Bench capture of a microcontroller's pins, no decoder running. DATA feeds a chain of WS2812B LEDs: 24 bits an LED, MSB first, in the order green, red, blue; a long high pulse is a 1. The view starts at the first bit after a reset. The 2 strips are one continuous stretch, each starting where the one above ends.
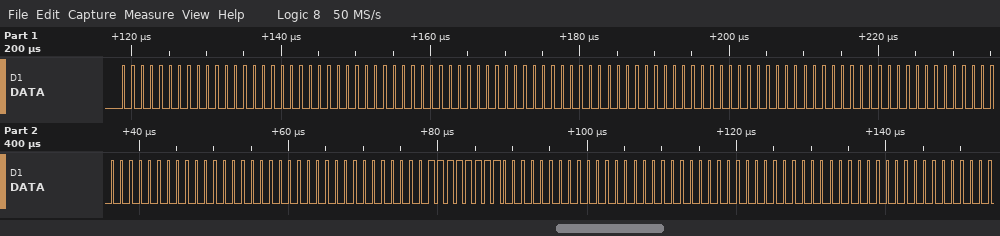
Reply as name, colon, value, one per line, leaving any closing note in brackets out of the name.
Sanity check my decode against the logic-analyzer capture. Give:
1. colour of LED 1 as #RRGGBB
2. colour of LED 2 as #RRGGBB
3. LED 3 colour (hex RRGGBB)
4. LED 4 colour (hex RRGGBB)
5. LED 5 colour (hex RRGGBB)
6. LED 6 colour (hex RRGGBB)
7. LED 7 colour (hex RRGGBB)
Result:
colour of LED 1 as #RRGGBB: #000000
colour of LED 2 as #RRGGBB: #000000
LED 3 colour: #000000
LED 4 colour: #000000
LED 5 colour: #000000
LED 6 colour: #FF0000
LED 7 colour: #000000
